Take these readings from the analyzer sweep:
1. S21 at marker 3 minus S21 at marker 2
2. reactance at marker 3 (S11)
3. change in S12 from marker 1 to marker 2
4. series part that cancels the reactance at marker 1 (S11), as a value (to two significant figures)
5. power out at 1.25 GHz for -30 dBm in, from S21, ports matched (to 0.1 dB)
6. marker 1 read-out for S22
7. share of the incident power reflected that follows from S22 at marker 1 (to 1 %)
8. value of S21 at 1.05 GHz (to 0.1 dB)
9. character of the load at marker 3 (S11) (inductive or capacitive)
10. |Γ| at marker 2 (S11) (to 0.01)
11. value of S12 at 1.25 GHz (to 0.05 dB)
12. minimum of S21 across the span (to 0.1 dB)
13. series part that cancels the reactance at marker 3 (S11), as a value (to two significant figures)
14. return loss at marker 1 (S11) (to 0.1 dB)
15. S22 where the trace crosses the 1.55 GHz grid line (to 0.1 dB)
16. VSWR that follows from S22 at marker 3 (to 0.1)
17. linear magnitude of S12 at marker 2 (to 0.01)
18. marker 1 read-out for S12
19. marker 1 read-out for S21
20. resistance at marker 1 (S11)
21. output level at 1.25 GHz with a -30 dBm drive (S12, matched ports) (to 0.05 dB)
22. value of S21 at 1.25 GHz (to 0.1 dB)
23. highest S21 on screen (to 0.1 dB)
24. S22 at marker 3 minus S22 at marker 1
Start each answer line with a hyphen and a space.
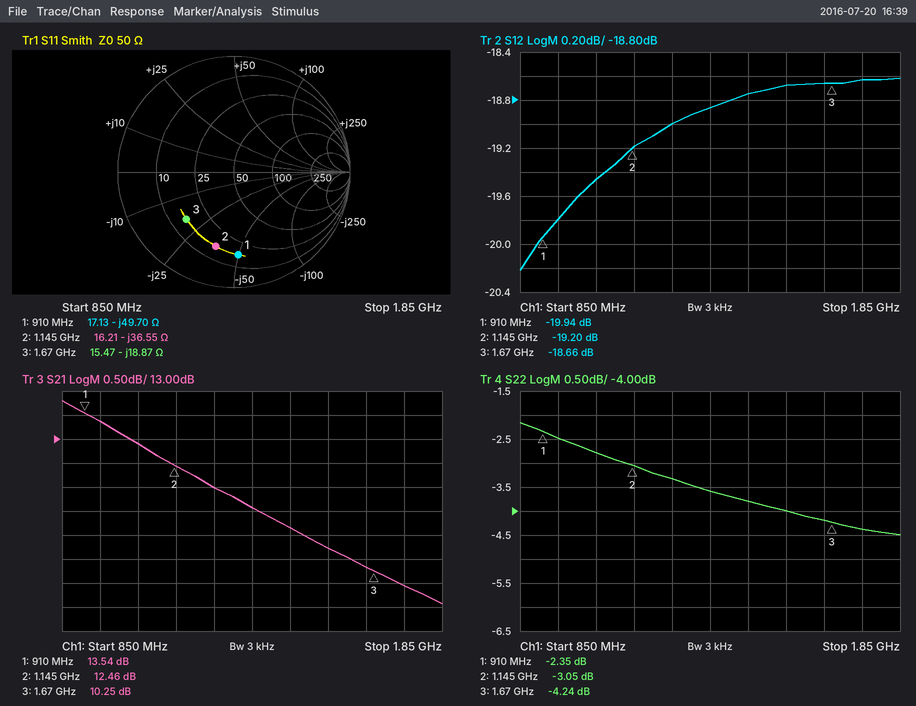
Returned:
- -2.21 dB
- -18.87 Ω
- 0.74 dB
- 8.7 nH
- -18.0 dBm
- -2.35 dB
- 58 %
- 12.9 dB
- capacitive
- 0.66
- -19.00 dB
- 9.6 dB
- 1.8 nH
- 2.9 dB
- -4.0 dB
- 4.2
- 0.11
- -19.94 dB
- 13.54 dB
- 17.13 Ω
- -49.00 dBm
- 12.0 dB
- 13.8 dB
- -1.89 dB
